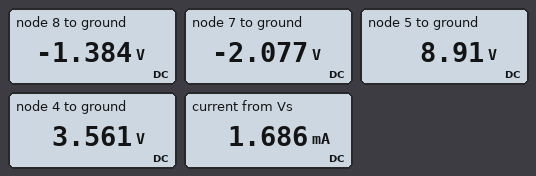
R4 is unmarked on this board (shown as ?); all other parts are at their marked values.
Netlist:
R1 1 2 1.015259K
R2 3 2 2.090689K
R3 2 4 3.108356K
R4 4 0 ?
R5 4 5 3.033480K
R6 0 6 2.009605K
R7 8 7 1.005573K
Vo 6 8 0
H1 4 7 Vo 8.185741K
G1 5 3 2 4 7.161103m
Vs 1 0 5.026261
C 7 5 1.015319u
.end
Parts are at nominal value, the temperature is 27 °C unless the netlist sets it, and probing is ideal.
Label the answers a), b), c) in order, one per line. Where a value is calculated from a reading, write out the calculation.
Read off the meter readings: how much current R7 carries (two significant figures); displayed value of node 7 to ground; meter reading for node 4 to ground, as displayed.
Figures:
a) (-1.384 V - (-2.077 V)) / 1.006 kΩ = 690 µA
b) -2.077 V
c) 3.561 V
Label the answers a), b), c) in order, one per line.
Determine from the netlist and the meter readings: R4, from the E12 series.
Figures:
a) 1.5 kΩ
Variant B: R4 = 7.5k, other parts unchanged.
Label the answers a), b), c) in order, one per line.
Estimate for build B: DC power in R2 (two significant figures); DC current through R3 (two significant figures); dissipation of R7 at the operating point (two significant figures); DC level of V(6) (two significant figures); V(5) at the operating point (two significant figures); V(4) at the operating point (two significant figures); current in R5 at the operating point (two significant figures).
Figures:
a) 230 µW
b) 15 µA
c) 1.1 mW
d) -2.1 V
e) 4.3 V
f) 5.3 V
g) 330 µA
